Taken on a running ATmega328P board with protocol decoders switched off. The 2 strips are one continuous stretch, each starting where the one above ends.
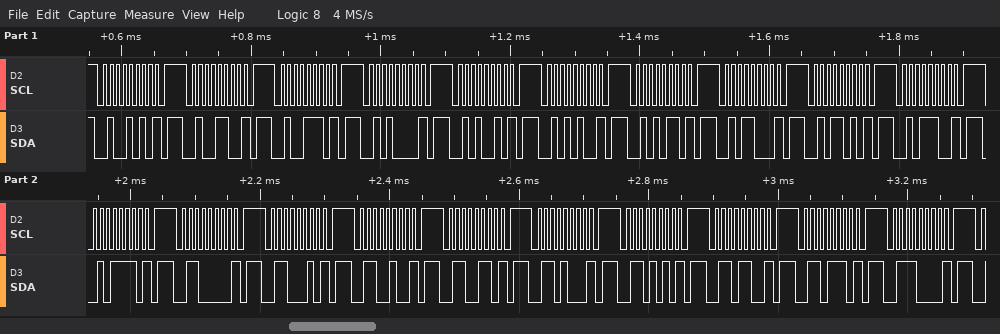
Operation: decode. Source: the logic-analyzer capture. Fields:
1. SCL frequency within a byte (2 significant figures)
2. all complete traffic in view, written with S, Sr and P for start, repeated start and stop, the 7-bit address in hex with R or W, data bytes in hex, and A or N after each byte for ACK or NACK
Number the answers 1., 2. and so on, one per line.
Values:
1. 100 kHz
2. S 25W N P S 26W N P S 27W N P S 28W N P S 29W N P S 2AW N P S 2BW N P S 2CW N P S 2DW N P S 2EW N P S 2FW N P S 30W N P S 31W N P S 32W N P S 33W N P S 34W N P S 35W N P S 36W N P S 37W N P S 38W N P
